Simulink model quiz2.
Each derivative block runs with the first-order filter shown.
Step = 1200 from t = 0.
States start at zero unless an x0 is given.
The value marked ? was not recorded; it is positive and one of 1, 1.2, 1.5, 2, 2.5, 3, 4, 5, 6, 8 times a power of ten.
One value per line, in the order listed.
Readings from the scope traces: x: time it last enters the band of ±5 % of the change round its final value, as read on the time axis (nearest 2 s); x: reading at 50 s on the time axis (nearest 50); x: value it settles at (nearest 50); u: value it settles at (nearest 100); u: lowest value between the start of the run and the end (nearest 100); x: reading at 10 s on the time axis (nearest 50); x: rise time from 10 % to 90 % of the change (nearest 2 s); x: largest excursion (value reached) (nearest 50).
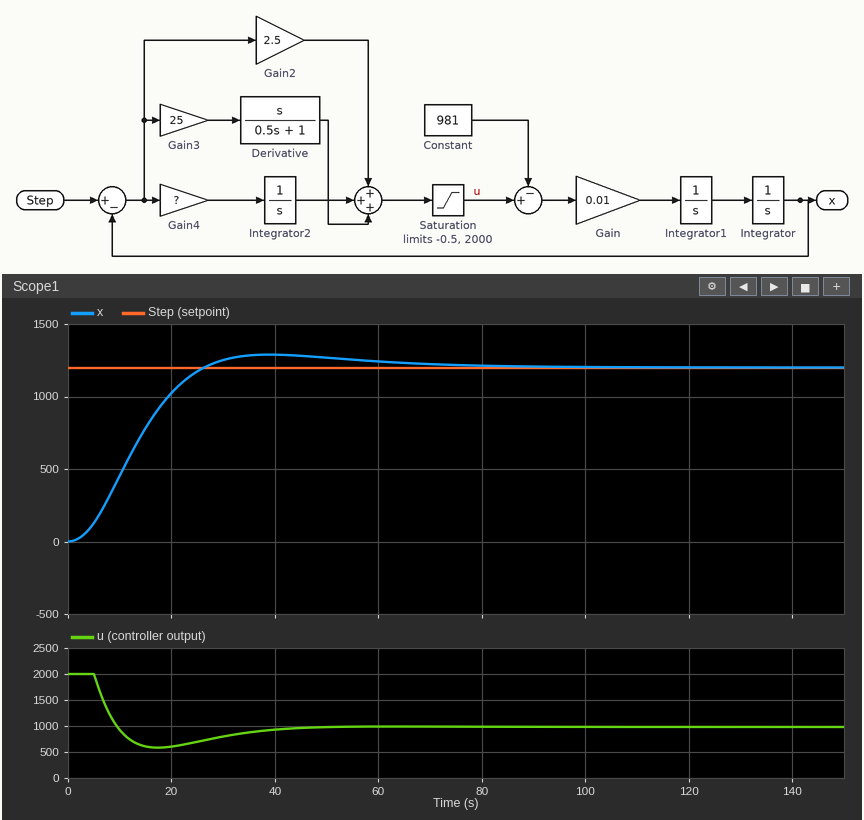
52 s
1250
1200
1000
600
450
16 s
1300
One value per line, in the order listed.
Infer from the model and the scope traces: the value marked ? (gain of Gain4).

0.08
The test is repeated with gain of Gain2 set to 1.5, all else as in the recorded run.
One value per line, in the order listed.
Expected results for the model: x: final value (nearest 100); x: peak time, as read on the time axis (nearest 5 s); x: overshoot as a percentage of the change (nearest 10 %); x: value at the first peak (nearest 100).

1200
50 s
20 %
1500
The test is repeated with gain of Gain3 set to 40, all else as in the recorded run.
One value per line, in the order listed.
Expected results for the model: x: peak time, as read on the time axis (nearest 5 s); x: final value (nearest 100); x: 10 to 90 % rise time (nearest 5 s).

60 s
1200
25 s
